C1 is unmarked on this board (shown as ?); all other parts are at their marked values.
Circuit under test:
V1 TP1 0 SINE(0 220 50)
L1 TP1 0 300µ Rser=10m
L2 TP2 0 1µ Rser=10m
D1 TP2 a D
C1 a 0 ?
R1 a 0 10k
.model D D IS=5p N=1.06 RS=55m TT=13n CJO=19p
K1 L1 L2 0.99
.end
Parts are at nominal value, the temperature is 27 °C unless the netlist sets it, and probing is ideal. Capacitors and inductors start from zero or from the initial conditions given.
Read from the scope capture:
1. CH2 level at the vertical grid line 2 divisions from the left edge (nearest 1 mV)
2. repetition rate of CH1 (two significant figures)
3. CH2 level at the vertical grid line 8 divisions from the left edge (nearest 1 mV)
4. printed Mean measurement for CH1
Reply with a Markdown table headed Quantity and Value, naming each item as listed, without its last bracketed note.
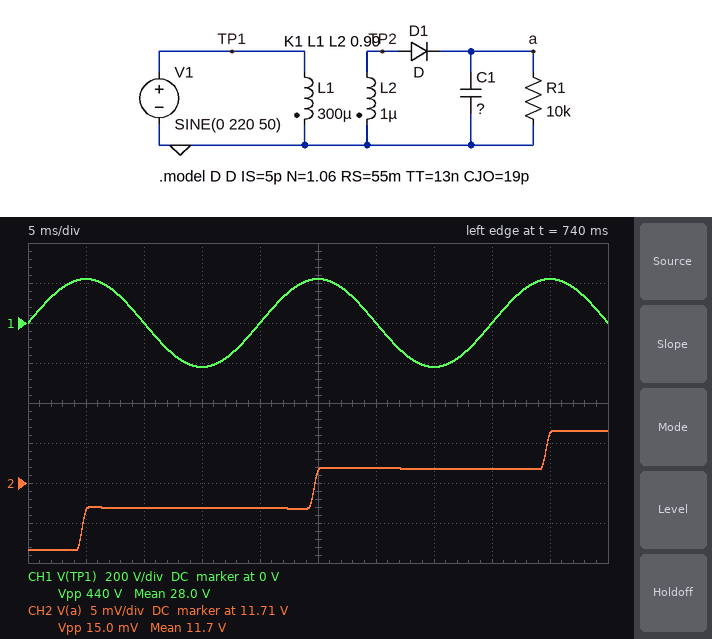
| Quantity | Value |
|---|---|
| CH2 level at the vertical grid line 2 divisions from the left edge | 11.702 V |
| repetition rate of CH1 | 50 Hz |
| CH2 level at the vertical grid line 8 divisions from the left edge | 11.707 V |
| printed Mean measurement for CH1 | 28.0 V |
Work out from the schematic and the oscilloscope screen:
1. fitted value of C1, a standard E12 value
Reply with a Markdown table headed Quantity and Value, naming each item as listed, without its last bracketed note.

| Quantity | Value |
|---|---|
| fitted value of C1, a standard E12 value | 150 mF |
